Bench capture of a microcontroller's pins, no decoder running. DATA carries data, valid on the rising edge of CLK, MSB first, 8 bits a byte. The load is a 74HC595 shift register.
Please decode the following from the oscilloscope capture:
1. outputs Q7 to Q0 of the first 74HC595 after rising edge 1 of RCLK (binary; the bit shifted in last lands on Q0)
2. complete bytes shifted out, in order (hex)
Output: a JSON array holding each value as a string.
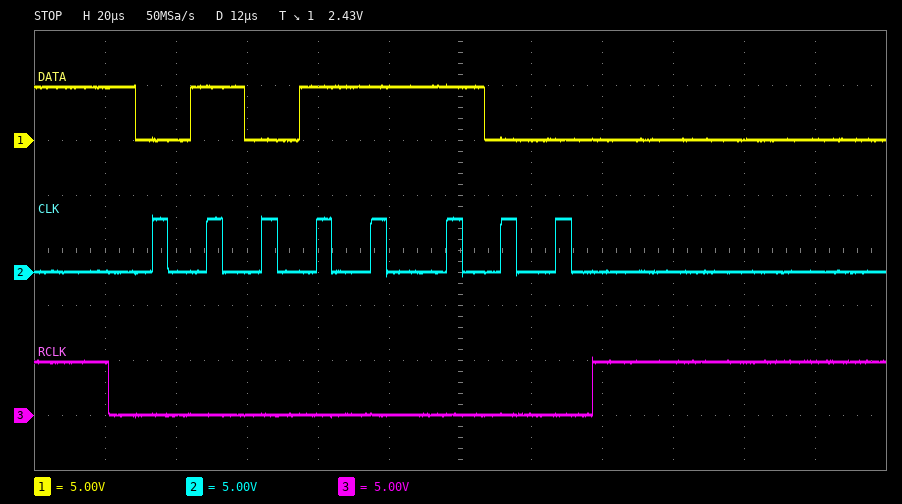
["01011100", "0x5C"]
